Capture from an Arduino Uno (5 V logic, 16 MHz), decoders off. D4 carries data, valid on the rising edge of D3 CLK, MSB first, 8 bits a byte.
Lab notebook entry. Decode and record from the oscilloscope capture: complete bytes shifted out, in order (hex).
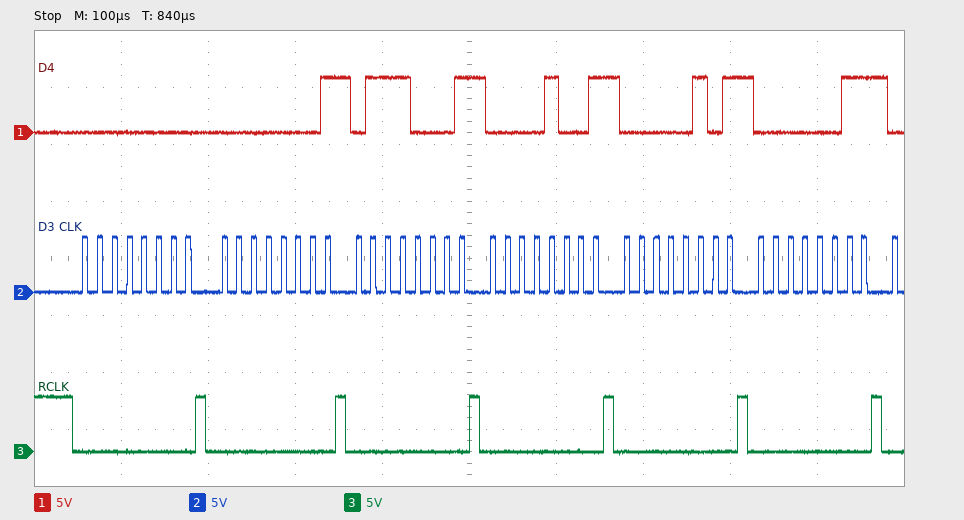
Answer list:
0x00 0x01 0x71 0x09 0x05 0x03
